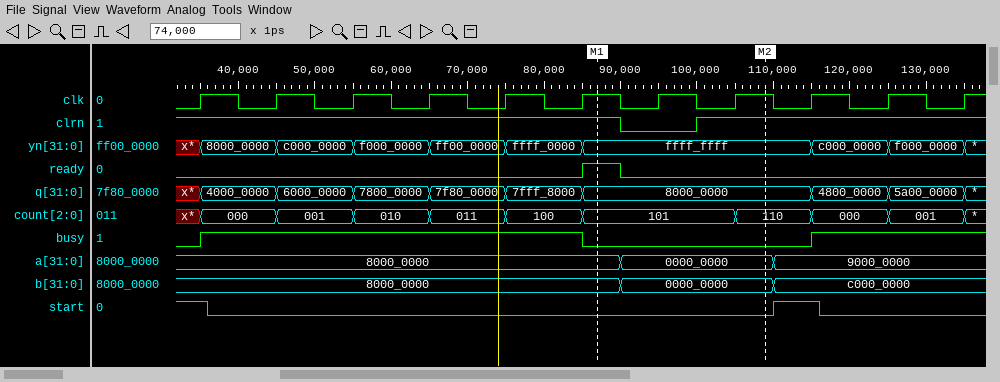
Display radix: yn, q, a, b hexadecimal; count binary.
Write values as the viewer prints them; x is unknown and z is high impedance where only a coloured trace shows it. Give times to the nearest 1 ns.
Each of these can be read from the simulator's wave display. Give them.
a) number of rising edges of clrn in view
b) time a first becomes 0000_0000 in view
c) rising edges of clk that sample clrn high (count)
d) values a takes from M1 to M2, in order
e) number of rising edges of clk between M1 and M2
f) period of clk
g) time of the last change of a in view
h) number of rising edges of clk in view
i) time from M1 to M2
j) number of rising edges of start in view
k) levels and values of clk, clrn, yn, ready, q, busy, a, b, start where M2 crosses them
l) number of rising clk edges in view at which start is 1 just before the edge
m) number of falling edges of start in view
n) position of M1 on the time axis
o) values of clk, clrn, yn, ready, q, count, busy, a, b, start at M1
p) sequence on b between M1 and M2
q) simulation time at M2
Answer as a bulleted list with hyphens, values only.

- 1
- 90 ns
- 10
- 8000_0000, 0000_0000
- 2
- 10 ns
- 110 ns
- 11
- 22 ns
- 1
- clk=1, clrn=1, yn=ffff_ffff, ready=0, q=8000_0000, busy=0, a=0000_0000, b=0000_0000, start=0
- 2
- 2
- 87 ns
- clk=1, clrn=1, yn=ffff_ffff, ready=1, q=8000_0000, count=101, busy=0, a=8000_0000, b=8000_0000, start=0
- 8000_0000, 0000_0000
- 109 ns
